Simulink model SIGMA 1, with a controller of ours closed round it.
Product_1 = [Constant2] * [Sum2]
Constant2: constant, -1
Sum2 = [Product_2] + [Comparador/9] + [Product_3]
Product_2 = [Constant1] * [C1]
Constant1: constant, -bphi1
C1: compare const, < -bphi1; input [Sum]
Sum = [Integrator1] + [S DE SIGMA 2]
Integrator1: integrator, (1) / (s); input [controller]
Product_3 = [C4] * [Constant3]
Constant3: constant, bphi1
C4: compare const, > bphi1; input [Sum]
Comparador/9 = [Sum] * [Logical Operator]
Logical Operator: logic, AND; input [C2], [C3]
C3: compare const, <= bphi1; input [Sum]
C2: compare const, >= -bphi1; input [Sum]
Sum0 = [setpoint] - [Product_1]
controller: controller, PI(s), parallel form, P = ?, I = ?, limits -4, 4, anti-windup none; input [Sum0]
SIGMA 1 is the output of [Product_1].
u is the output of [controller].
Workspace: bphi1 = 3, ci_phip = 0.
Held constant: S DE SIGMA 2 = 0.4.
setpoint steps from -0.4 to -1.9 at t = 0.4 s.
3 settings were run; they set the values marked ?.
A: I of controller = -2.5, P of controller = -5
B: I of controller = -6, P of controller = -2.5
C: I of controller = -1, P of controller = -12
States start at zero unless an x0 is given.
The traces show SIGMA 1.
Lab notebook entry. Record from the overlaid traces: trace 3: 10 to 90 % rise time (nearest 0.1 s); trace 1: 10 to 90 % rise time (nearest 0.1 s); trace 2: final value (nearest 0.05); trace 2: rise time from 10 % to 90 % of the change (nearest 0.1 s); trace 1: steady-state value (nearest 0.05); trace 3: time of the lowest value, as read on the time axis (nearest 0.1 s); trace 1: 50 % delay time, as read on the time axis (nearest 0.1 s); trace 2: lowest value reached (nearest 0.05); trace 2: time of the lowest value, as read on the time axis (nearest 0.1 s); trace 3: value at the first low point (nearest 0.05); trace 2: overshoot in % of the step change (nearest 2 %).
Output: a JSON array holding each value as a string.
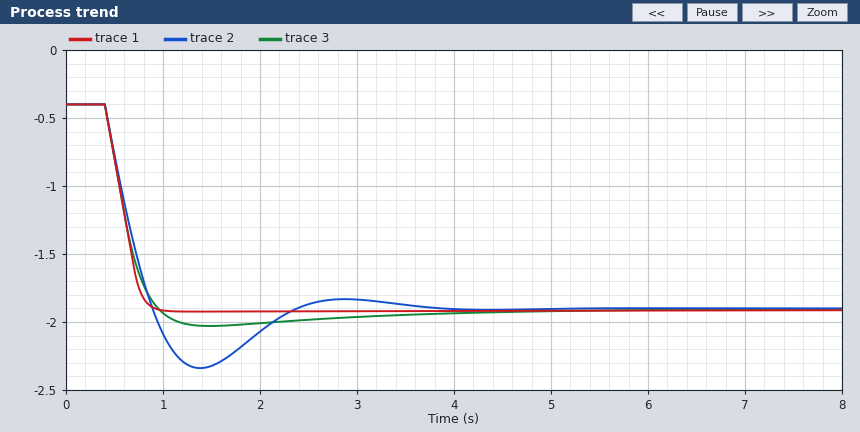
["0.4 s", "0.3 s", "-1.90", "0.4 s", "-1.90", "1.5 s", "0.6 s", "-2.35", "1.4 s", "-2.05", "30 %"]
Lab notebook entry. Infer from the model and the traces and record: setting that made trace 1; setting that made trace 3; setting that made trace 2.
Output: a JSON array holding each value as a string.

["C", "A", "B"]
